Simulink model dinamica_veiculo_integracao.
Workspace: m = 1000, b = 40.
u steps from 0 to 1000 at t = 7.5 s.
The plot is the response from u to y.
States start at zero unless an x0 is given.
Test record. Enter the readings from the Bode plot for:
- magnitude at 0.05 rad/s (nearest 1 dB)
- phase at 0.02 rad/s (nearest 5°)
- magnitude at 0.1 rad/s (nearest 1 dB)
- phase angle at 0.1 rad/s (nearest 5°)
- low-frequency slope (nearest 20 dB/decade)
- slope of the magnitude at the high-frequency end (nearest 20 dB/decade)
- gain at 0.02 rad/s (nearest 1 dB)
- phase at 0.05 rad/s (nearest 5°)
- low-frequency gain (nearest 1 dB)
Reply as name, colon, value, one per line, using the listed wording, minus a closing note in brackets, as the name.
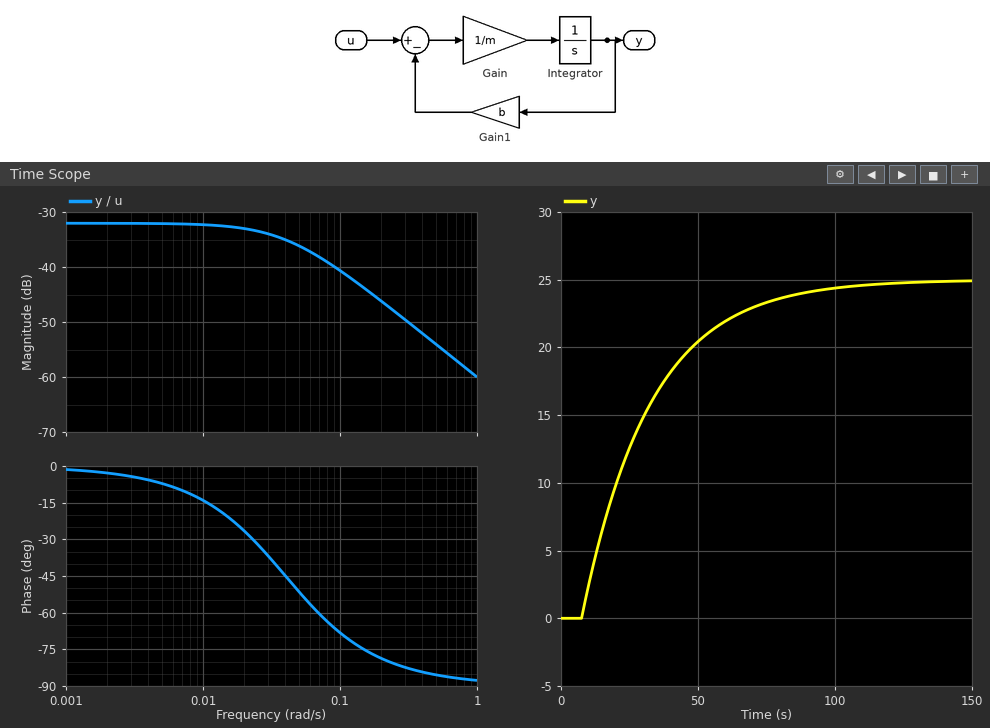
magnitude at 0.05 rad/s: -36 dB
phase at 0.02 rad/s: -25°
magnitude at 0.1 rad/s: -41 dB
phase angle at 0.1 rad/s: -70°
low-frequency slope: 0 dB/decade
slope of the magnitude at the high-frequency end: -20 dB/decade
gain at 0.02 rad/s: -33 dB
phase at 0.05 rad/s: -50°
low-frequency gain: -32 dB
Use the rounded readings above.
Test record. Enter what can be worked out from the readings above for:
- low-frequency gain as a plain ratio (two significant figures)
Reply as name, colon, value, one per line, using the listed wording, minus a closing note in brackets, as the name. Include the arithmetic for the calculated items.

low-frequency gain as a plain ratio: 10^(-32 / 20) = 0.025
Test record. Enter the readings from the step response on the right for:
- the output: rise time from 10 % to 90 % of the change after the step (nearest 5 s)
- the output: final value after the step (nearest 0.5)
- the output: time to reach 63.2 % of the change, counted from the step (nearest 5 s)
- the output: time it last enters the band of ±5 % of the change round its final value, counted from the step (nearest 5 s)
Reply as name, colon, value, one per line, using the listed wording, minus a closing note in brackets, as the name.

the output: rise time from 10 % to 90 % of the change after the step: 55 s
the output: final value after the step: 25.0
the output: time to reach 63.2 % of the change, counted from the step: 25 s
the output: time it last enters the band of ±5 % of the change round its final value, counted from the step: 75 s
